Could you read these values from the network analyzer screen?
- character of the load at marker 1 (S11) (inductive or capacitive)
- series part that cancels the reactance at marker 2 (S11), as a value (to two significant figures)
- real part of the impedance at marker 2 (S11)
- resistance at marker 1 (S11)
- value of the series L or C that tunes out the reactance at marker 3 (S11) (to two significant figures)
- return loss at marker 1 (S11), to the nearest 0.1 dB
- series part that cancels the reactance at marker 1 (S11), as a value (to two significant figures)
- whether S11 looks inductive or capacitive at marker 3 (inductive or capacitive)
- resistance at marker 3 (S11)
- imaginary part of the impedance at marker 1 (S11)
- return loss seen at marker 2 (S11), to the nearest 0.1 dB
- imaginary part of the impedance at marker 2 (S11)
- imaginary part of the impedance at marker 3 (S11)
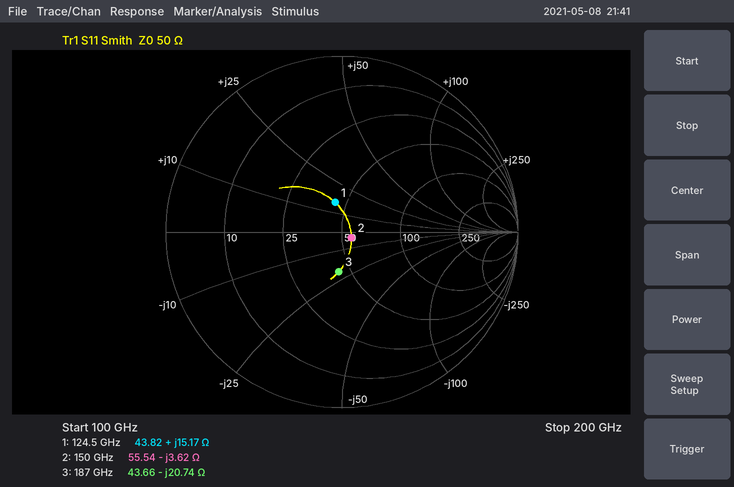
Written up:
inductive
3.8 pH
55.54 Ω
43.82 Ω
18 pH
15.3 dB
84 fF
capacitive
43.66 Ω
+15.17 Ω
24.1 dB
-3.62 Ω
-20.74 Ω
